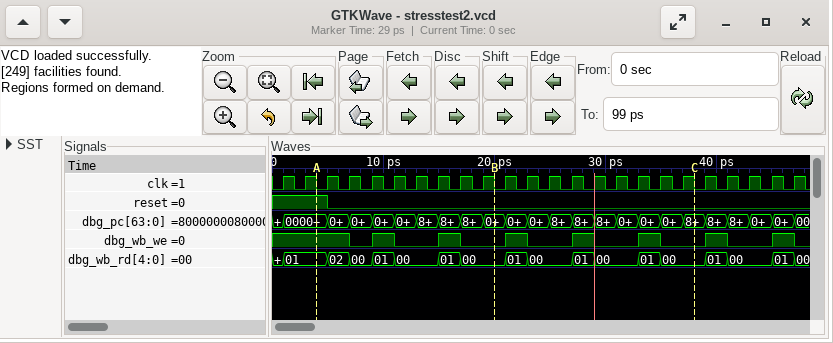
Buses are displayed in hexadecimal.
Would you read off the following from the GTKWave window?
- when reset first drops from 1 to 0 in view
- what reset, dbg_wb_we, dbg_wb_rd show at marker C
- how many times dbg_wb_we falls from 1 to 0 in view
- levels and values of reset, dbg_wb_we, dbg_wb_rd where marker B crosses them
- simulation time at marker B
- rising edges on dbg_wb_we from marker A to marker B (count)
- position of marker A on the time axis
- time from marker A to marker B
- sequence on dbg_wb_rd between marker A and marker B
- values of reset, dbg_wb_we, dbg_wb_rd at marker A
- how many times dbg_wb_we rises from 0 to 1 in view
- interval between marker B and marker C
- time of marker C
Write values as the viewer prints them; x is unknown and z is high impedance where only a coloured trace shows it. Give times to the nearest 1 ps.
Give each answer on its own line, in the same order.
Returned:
5 ps
reset=0, dbg_wb_we=0, dbg_wb_rd=00
8
reset=0, dbg_wb_we=0, dbg_wb_rd=00
20 ps
2
4 ps
16 ps
01, 02, 00, 01, 00, 01, 00
reset=1, dbg_wb_we=1, dbg_wb_rd=01
7
18 ps
38 ps
